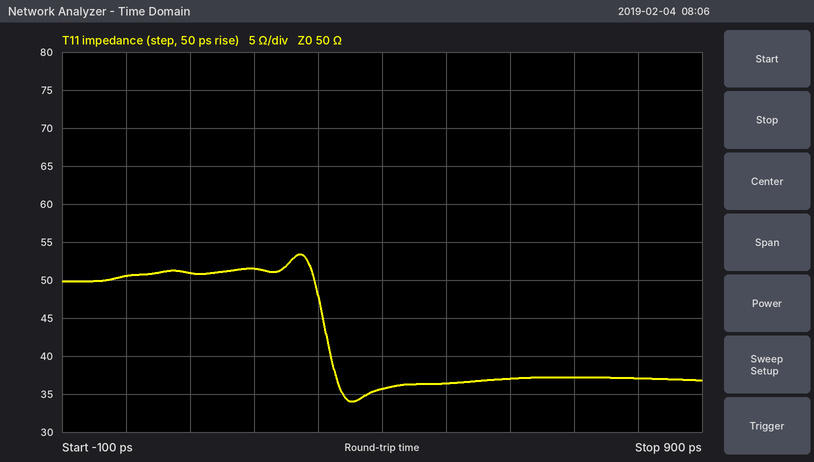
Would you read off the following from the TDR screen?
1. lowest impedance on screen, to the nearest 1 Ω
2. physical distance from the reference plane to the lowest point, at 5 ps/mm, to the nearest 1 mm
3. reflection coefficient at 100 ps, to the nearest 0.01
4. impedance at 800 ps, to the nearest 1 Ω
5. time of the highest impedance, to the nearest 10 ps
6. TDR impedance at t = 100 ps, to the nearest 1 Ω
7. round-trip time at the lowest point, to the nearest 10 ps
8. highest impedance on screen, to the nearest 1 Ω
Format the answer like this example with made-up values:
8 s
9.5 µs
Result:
34 Ω
35 mm
+0.01
37 Ω
270 ps
51 Ω
350 ps
53 Ω
